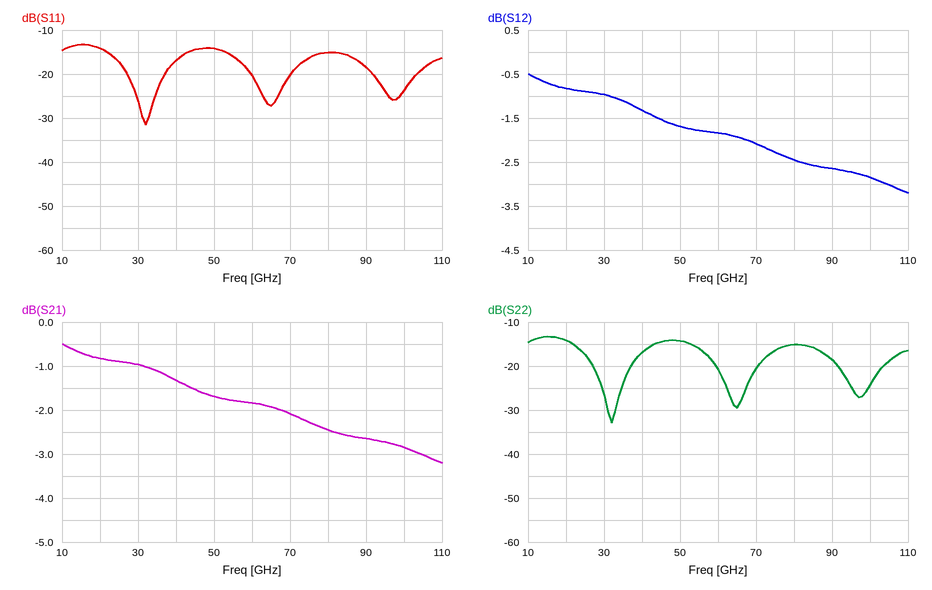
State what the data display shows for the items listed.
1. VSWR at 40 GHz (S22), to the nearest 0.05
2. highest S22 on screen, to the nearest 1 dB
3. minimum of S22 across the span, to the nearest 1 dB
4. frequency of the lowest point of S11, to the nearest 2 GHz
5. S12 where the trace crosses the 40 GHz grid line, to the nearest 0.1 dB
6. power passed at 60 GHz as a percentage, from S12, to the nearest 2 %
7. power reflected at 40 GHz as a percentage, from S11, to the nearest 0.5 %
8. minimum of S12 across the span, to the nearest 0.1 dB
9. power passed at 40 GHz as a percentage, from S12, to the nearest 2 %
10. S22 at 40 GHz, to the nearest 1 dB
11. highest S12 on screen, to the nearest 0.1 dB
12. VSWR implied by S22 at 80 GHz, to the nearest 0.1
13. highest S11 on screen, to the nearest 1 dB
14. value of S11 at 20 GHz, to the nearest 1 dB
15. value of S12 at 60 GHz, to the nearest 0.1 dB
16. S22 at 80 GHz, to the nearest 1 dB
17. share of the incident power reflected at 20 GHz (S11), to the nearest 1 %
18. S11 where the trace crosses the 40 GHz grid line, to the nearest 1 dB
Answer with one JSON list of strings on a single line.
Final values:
["1.35", "-13 dB", "-33 dB", "32 GHz", "-1.3 dB", "66 %", "2.0 %", "-3.2 dB", "74 %", "-17 dB", "-0.5 dB", "1.4", "-13 dB", "-14 dB", "-1.8 dB", "-15 dB", "4 %", "-17 dB"]
